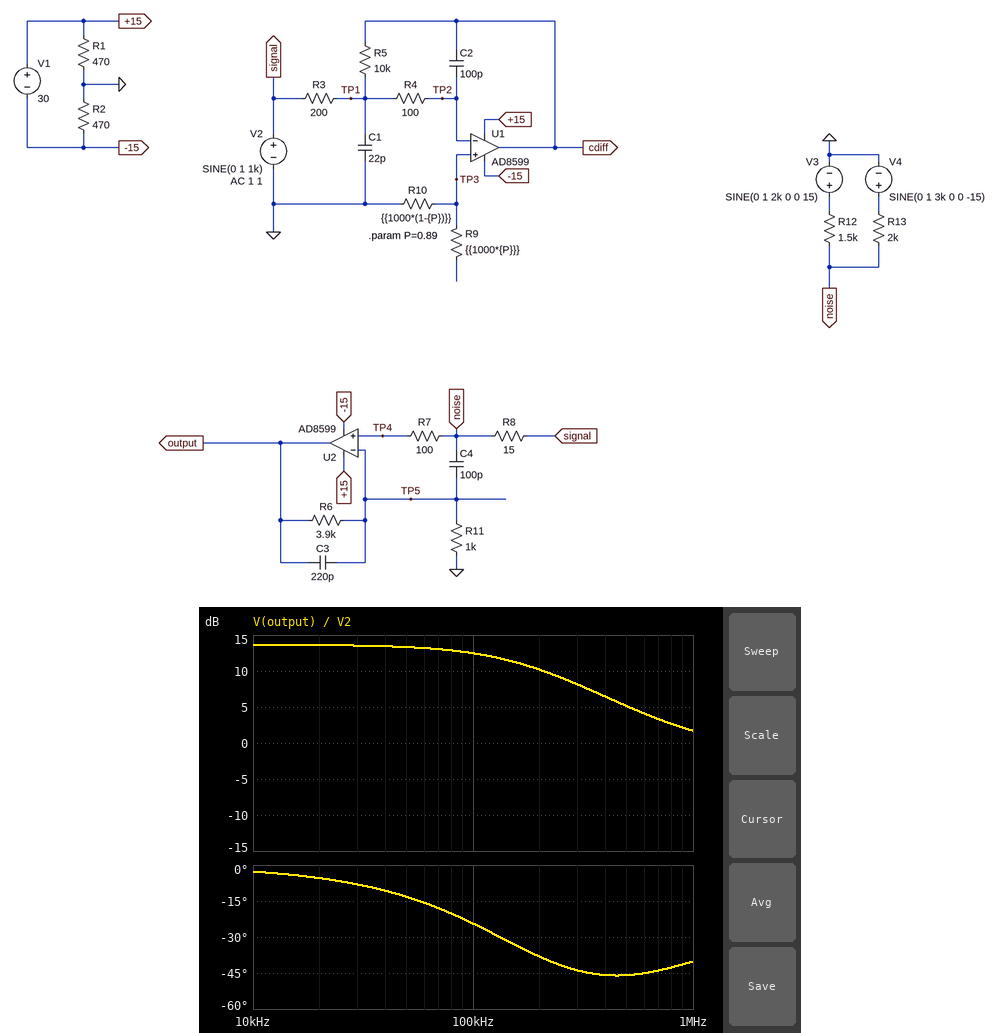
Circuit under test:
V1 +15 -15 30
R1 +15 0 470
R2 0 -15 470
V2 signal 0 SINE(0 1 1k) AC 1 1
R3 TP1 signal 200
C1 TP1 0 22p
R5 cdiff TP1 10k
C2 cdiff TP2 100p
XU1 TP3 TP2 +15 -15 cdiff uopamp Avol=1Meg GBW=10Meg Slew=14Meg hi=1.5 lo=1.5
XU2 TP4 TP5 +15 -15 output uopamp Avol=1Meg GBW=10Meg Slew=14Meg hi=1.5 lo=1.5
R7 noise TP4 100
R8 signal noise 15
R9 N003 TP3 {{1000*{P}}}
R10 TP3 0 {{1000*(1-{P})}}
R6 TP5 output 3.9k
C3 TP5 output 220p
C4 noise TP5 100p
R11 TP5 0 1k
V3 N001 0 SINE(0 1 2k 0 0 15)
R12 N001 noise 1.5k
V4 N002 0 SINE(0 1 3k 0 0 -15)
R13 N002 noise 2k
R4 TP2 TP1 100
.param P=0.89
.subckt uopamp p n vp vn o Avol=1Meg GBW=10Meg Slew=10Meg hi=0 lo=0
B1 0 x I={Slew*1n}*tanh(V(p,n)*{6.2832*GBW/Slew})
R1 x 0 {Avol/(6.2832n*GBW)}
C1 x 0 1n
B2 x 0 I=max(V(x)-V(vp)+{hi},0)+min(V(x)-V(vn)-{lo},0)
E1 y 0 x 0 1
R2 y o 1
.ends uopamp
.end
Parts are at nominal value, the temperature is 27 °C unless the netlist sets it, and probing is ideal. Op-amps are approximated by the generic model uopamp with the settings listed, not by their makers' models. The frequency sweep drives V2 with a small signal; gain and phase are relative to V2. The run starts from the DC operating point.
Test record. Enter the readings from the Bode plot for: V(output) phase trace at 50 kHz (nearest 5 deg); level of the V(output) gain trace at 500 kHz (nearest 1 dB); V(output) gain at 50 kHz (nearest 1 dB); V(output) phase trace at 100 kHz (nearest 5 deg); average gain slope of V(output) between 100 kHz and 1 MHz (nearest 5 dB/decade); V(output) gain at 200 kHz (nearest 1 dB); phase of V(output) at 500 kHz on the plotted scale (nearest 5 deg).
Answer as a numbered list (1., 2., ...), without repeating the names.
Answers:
1. -15 deg
2. 5 dB
3. 13 dB
4. -25 deg
5. -10 dB/decade
6. 10 dB
7. -45 deg
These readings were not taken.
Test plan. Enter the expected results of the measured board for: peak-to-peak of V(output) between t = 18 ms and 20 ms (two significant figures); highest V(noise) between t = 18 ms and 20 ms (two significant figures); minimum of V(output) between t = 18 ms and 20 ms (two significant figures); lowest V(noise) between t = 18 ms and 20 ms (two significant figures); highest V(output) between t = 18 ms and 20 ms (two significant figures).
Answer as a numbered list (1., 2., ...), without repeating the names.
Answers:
1. 9.6 V
2. 970 mV
3. -4.8 V
4. -980 mV
5. 4.8 V
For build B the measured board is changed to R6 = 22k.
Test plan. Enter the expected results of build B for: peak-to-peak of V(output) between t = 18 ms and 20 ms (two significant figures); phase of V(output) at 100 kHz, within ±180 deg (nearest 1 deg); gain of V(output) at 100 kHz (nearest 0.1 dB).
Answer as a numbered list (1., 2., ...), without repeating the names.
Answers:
1. 27 V
2. -66 deg
3. 16.5 dB
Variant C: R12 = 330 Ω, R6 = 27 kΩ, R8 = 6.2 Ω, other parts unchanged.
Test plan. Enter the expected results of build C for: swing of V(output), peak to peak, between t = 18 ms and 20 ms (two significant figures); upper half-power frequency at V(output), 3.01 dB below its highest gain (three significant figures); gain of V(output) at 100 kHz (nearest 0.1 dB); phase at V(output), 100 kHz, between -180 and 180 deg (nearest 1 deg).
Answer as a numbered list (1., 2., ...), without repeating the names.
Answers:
1. 27 V
2. 25.0 kHz
3. 16.5 dB
4. -69 deg
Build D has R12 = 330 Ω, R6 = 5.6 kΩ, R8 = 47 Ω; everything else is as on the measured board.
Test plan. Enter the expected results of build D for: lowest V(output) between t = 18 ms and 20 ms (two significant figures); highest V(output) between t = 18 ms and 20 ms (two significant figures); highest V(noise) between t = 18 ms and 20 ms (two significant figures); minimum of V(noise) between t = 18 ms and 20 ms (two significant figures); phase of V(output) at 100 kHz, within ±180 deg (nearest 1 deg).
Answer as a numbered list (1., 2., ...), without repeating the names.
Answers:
1. -5.9 V
2. 5.6 V
3. 850 mV
4. -900 mV
5. -34 deg
